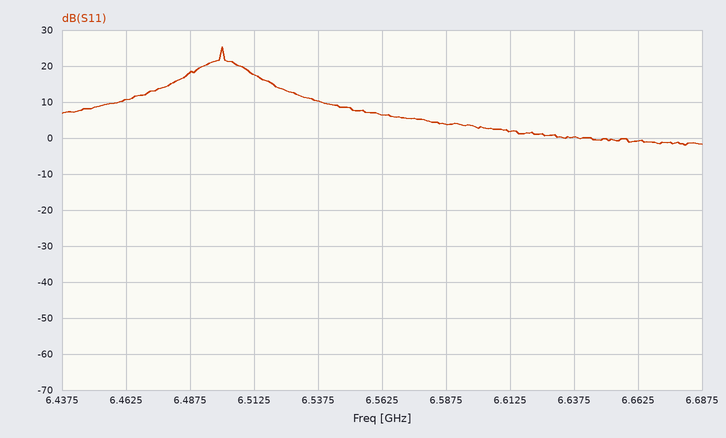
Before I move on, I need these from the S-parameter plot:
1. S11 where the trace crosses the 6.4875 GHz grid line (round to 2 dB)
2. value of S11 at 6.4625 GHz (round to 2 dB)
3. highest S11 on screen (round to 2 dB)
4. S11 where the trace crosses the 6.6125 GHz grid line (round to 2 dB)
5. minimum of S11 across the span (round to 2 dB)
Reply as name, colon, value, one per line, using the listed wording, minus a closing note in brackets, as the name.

S11 where the trace crosses the 6.4875 GHz grid line: 18 dB
value of S11 at 6.4625 GHz: 10 dB
highest S11 on screen: 26 dB
S11 where the trace crosses the 6.6125 GHz grid line: 2 dB
minimum of S11 across the span: -2 dB
